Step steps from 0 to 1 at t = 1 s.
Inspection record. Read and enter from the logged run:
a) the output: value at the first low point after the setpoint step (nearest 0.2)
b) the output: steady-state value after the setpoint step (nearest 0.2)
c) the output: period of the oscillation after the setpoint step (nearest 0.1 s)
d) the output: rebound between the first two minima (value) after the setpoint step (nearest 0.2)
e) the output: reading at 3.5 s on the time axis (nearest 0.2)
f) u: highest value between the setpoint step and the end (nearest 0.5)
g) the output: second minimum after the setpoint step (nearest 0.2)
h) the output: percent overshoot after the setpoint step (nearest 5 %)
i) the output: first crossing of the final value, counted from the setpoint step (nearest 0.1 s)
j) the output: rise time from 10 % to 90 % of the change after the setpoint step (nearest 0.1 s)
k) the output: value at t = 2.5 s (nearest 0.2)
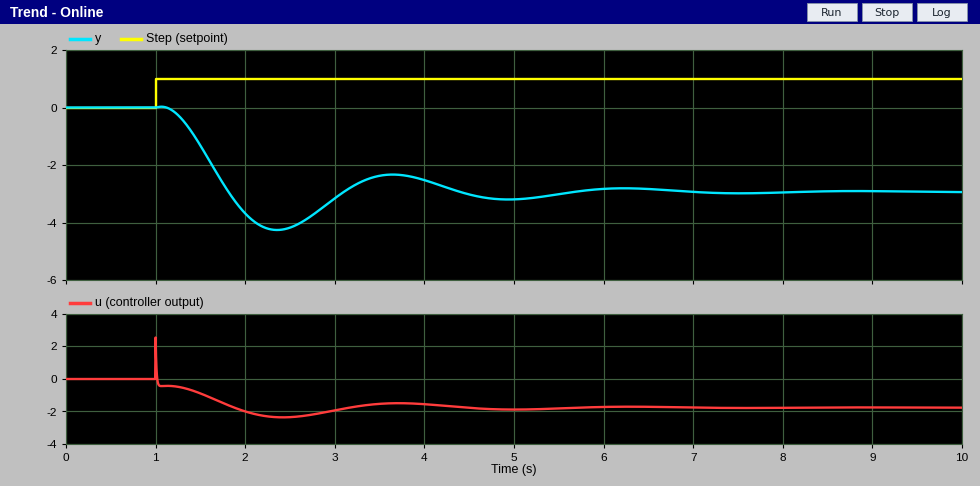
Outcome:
-4.2
-3.0
2.6 s
-2.4
-2.4
2.5
-3.2
45 %
0.8 s
0.5 s
-4.2
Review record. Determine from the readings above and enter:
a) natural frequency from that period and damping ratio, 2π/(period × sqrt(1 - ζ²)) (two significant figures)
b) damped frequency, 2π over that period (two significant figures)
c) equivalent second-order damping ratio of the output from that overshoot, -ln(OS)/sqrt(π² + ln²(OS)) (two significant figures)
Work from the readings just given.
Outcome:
2.5 rad/s
2.4 rad/s
0.25
